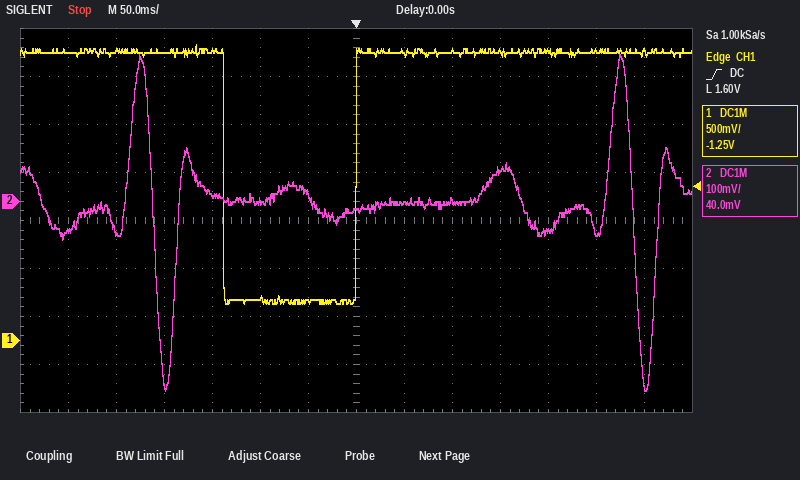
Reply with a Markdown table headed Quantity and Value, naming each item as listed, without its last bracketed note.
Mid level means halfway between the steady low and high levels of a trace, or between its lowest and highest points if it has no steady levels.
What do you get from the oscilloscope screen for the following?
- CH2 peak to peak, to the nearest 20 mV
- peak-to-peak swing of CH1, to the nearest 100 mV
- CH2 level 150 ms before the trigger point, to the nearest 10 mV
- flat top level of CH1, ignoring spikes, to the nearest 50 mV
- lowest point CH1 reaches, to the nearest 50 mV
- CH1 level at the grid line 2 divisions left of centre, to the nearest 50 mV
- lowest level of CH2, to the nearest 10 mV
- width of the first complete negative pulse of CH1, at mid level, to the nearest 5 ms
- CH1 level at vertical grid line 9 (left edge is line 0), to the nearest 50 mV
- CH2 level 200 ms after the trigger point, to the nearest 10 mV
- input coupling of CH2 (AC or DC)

| Quantity | Value |
|---|---|
| CH2 peak to peak, to the nearest 20 mV | 700 mV |
| peak-to-peak swing of CH1, to the nearest 100 mV | 2.70 V |
| CH2 level 150 ms before the trigger point, to the nearest 10 mV | 10 mV |
| flat top level of CH1, ignoring spikes, to the nearest 50 mV | 3.00 V |
| lowest point CH1 reaches, to the nearest 50 mV | 400 mV |
| CH1 level at the grid line 2 divisions left of centre, to the nearest 50 mV | 450 mV |
| lowest level of CH2, to the nearest 10 mV | -390 mV |
| width of the first complete negative pulse of CH1, at mid level, to the nearest 5 ms | 140 ms |
| CH1 level at vertical grid line 9 (left edge is line 0), to the nearest 50 mV | 3.00 V |
| CH2 level 200 ms after the trigger point, to the nearest 10 mV | -60 mV |
| input coupling of CH2 | DC |
